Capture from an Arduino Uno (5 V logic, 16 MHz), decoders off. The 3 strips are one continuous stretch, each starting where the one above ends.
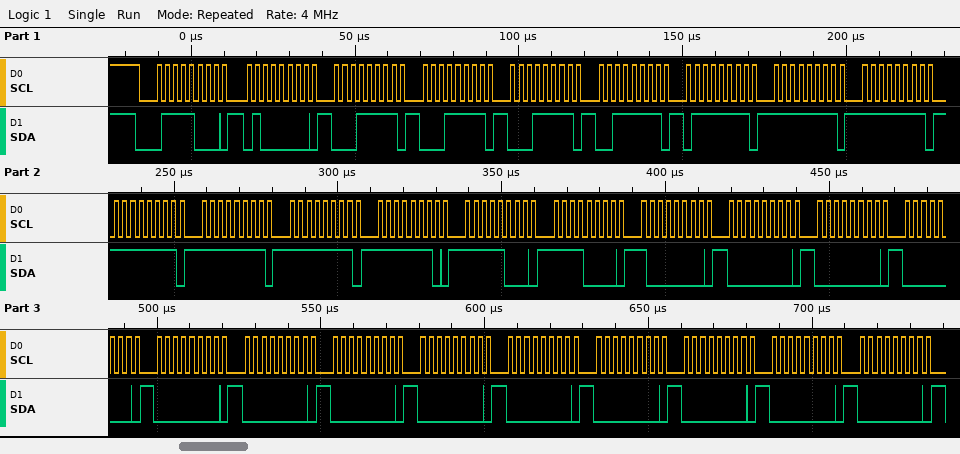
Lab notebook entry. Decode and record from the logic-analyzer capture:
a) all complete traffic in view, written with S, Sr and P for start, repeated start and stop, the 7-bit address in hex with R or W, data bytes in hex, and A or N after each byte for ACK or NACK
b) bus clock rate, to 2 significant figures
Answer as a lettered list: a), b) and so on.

a) S 3CW A 40 A 1F A 1F A 1F A 3F A 7F A FF A FF A FF A FF A FF A FE A F8 A F0 A 80 A 00 A 00 A 00 A 00 A 00 A 00 A 00 A 00 A 00 A 00 A 00 A 00 A
b) 400 kHz
